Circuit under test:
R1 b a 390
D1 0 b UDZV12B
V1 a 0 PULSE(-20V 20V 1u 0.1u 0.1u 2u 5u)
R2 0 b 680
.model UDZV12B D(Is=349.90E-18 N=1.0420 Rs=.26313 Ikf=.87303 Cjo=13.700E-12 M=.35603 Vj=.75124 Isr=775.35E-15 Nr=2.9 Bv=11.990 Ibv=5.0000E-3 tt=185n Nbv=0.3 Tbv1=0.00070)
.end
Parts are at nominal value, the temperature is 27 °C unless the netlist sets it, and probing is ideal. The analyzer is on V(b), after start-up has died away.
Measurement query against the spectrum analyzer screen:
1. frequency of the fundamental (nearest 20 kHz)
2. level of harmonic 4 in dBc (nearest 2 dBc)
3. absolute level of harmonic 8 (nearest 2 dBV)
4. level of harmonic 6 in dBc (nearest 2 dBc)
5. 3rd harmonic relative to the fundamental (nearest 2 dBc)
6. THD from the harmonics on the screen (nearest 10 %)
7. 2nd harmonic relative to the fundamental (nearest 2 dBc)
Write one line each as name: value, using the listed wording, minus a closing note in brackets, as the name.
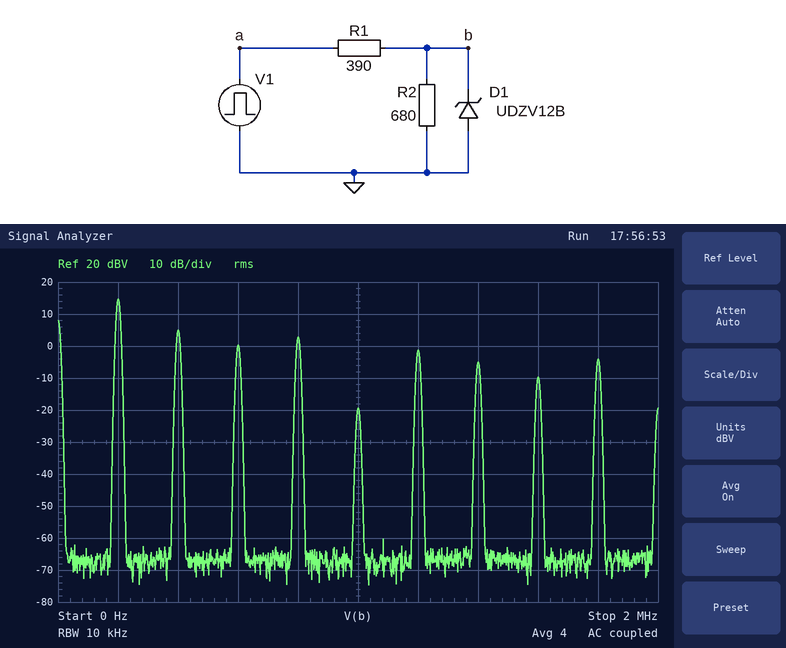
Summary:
frequency of the fundamental: 200 kHz
level of harmonic 4 in dBc: -12 dBc
absolute level of harmonic 8: -10 dBV
level of harmonic 6 in dBc: -16 dBc
3rd harmonic relative to the fundamental: -14 dBc
THD from the harmonics on the screen: 50 %
2nd harmonic relative to the fundamental: -10 dBc
